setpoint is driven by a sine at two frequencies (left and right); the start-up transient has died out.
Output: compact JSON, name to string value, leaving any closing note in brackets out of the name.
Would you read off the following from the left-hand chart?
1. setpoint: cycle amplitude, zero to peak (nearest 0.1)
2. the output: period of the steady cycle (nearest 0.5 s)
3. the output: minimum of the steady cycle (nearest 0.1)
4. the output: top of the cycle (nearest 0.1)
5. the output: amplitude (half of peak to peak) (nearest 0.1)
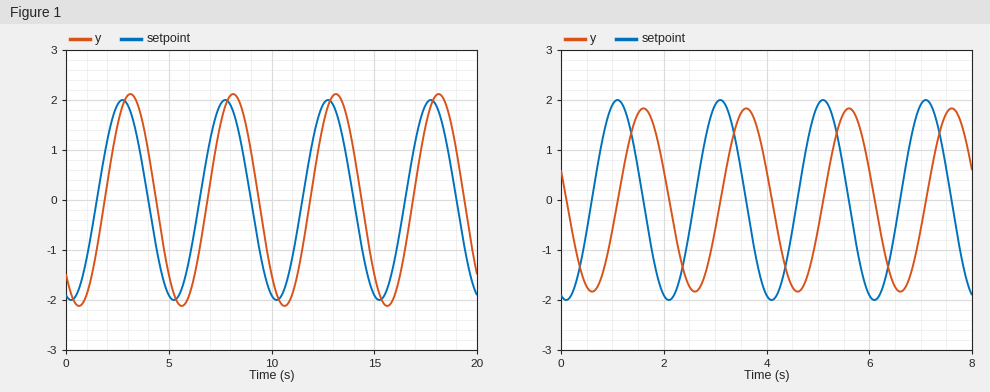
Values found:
{"setpoint: cycle amplitude, zero to peak": "2.0", "the output: period of the steady cycle": "5.0 s", "the output: minimum of the steady cycle": "-2.1", "the output: top of the cycle": "2.1", "the output: amplitude (half of peak to peak)": "2.1"}
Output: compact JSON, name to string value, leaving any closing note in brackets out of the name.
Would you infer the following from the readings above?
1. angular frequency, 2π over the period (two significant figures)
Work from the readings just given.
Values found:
{"angular frequency, 2π over the period": "1.3 rad/s"}
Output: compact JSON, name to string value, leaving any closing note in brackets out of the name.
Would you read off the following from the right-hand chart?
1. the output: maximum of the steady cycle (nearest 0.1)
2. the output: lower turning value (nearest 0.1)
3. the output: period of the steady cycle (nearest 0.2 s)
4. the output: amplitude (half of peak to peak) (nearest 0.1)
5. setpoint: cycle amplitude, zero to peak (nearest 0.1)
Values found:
{"the output: maximum of the steady cycle": "1.8", "the output: lower turning value": "-1.8", "the output: period of the steady cycle": "2.0 s", "the output: amplitude (half of peak to peak)": "1.8", "setpoint: cycle amplitude, zero to peak": "2.0"}
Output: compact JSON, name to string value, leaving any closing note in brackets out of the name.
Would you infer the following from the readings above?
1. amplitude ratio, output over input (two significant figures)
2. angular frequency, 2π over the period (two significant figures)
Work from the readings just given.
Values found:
{"amplitude ratio, output over input": "0.90", "angular frequency, 2π over the period": "3.1 rad/s"}
